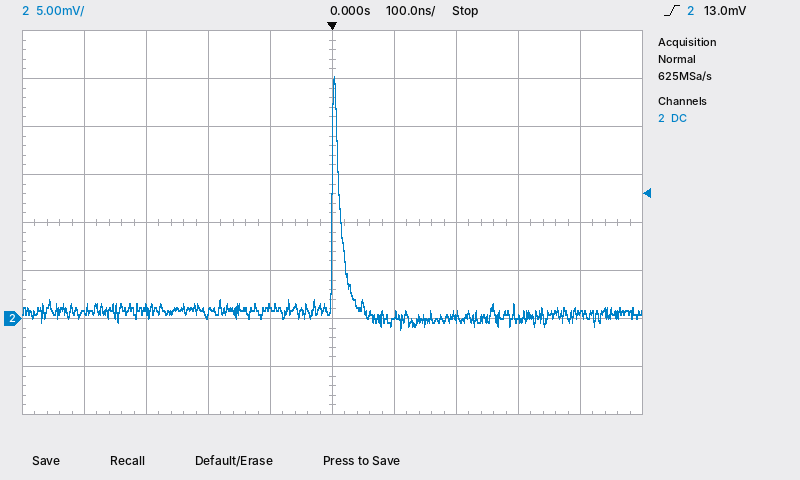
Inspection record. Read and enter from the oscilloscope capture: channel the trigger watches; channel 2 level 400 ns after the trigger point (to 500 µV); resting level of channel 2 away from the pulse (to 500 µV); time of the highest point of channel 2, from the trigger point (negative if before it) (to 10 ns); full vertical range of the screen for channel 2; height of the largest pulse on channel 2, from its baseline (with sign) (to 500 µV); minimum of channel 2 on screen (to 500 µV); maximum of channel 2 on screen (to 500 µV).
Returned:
channel 2
500 µV
500 µV
0 ns
40 mV
+24.5 mV
-1.0 mV
25.0 mV
